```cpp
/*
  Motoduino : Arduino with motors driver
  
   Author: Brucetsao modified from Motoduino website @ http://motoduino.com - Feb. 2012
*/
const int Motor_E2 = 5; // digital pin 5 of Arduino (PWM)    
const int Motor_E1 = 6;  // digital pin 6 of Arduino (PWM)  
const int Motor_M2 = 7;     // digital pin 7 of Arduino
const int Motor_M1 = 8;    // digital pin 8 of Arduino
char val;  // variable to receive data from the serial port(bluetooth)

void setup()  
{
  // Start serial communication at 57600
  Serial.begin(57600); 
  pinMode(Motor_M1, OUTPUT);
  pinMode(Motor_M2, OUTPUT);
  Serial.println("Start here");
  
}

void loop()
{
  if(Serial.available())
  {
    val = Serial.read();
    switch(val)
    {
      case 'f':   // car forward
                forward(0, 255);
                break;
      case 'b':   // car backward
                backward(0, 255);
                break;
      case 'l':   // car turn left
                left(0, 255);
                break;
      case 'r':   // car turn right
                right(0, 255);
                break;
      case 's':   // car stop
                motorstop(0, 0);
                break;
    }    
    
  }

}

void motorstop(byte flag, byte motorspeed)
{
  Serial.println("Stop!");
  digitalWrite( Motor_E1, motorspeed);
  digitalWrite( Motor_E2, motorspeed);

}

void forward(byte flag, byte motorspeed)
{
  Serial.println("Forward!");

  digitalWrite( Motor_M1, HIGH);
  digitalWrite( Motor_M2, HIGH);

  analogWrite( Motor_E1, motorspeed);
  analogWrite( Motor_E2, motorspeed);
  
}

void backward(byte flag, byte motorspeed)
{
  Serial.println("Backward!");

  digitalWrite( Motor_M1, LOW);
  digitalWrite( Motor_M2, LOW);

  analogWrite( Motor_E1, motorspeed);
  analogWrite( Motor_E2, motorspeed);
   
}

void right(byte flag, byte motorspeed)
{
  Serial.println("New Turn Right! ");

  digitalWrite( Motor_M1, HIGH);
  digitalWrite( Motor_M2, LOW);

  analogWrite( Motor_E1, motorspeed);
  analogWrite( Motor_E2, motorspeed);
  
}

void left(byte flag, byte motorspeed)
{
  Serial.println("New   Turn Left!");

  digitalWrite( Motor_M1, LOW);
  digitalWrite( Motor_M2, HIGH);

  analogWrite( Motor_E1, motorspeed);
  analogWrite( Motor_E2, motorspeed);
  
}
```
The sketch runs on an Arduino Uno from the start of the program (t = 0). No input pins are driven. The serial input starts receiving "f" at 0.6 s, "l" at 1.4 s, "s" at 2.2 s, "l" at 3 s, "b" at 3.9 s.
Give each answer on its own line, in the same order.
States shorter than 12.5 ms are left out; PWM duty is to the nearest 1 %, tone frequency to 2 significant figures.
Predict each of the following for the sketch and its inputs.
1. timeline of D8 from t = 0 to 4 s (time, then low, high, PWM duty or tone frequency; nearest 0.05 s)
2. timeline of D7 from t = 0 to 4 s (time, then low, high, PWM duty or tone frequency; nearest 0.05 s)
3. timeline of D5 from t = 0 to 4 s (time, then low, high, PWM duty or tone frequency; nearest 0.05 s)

0 s low; 0.6 s high; 1.4 s low
0 s low; 0.6 s high; 3.9 s low
0.6 s high; 2.2 s low; 3 s high
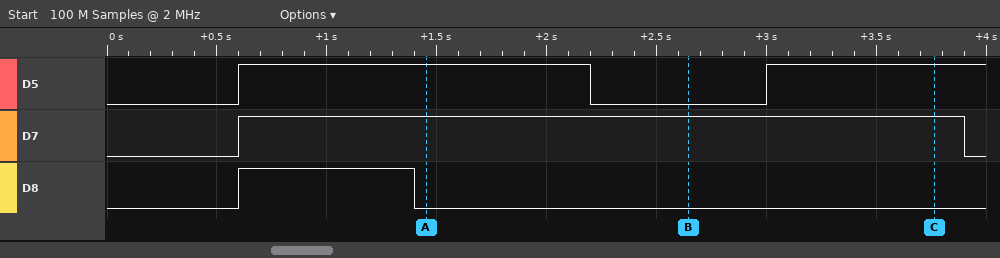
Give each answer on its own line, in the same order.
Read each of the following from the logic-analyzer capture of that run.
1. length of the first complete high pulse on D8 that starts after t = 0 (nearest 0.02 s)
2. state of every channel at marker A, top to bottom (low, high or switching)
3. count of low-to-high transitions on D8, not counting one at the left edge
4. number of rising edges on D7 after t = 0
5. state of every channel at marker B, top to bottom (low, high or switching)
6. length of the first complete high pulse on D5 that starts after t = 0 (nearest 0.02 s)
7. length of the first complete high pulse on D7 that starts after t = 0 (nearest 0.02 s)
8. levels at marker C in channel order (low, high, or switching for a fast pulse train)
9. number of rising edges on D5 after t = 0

0.80 s
D5 high, D7 high, D8 low
1
1
D5 low, D7 high, D8 low
1.60 s
3.30 s
D5 high, D7 high, D8 low
2
